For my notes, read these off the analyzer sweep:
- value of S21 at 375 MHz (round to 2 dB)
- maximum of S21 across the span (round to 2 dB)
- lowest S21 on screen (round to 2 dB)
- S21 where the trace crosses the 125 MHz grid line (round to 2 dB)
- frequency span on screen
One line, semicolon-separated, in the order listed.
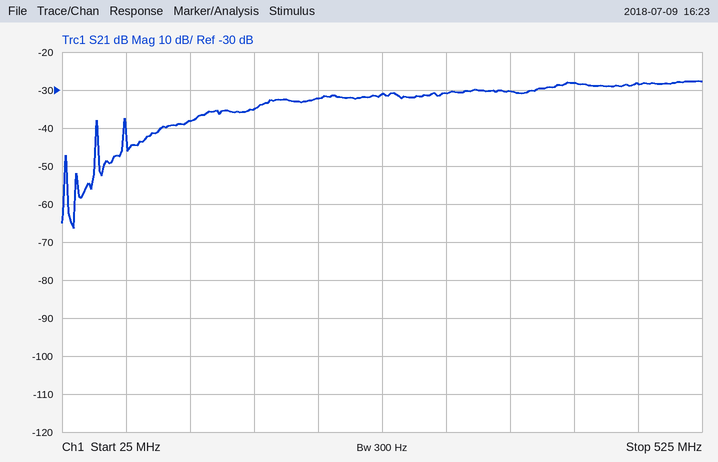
-30 dB; -28 dB; -66 dB; -38 dB; 500 MHz
